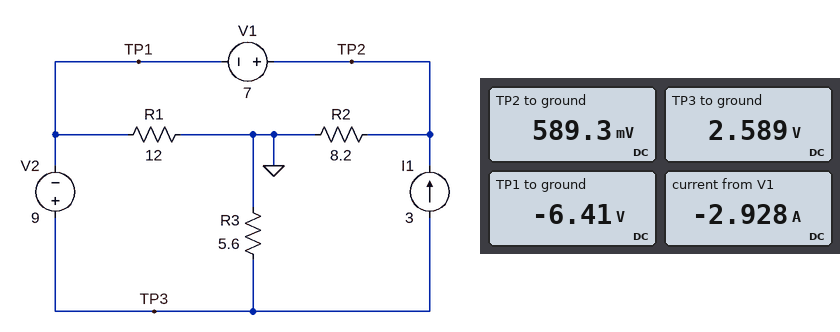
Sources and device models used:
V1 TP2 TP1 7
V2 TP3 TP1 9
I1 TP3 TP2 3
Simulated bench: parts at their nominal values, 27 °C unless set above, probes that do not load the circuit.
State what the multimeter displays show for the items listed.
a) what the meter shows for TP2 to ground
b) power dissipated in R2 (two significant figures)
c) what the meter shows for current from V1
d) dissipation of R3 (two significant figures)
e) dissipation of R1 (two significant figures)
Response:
589.3 mV
42 mW
-2.928 A
1.2 W
3.4 W
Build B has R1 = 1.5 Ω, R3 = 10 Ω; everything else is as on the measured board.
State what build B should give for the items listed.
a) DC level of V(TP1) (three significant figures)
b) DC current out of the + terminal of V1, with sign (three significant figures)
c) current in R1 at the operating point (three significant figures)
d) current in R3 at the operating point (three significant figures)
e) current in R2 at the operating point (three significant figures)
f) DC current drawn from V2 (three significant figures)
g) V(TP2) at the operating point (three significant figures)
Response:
-1.97 V
-2.39 A
1.32 A
703 mA
613 mA
3.70 A
5.03 V
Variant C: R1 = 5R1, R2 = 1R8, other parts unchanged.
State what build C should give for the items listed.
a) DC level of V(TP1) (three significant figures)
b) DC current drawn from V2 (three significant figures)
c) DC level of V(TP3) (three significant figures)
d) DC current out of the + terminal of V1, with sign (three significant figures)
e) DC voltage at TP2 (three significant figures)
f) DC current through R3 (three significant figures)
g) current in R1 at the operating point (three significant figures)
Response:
-5.91 V
3.55 A
3.09 V
-2.39 A
1.09 V
552 mA
1.16 A
